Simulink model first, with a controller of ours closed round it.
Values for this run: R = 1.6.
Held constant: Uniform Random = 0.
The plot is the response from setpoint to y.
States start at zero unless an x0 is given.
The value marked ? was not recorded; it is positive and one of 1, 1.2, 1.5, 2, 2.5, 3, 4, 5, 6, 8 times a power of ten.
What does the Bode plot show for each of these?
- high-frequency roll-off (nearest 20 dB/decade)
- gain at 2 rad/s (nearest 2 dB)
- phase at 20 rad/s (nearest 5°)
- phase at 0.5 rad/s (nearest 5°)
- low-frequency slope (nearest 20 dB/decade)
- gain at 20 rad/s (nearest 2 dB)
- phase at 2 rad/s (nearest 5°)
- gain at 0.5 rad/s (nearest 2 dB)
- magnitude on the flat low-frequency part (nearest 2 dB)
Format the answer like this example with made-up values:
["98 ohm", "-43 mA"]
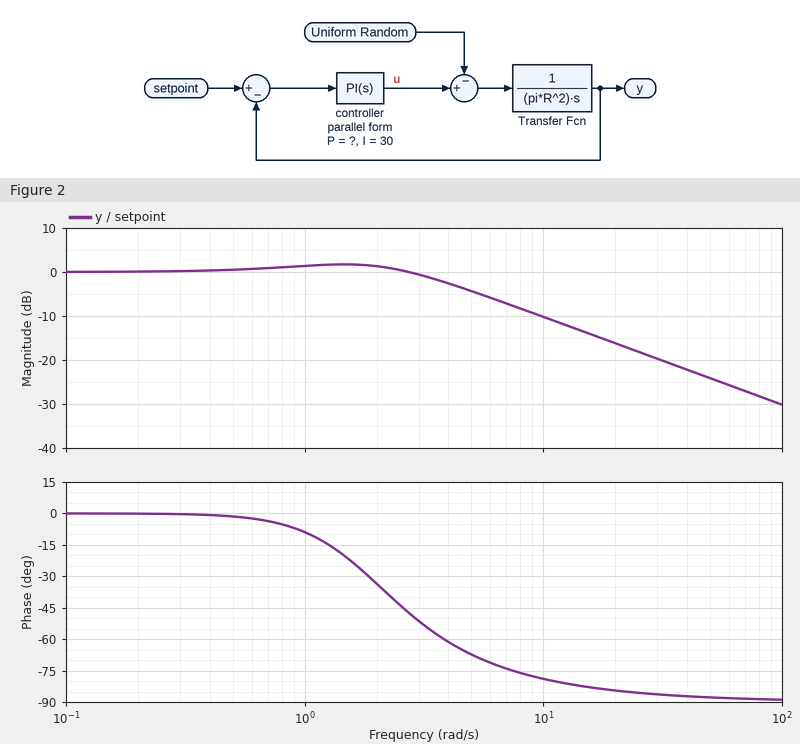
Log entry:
["-20 dB/decade", "2 dB", "-85°", "0°", "0 dB/decade", "-16 dB", "-35°", "0 dB", "0 dB"]
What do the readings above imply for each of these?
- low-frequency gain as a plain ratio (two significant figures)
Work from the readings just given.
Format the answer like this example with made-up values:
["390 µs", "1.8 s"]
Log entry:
["1.0"]
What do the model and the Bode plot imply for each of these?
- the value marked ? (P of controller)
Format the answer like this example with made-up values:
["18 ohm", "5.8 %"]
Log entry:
["25"]
